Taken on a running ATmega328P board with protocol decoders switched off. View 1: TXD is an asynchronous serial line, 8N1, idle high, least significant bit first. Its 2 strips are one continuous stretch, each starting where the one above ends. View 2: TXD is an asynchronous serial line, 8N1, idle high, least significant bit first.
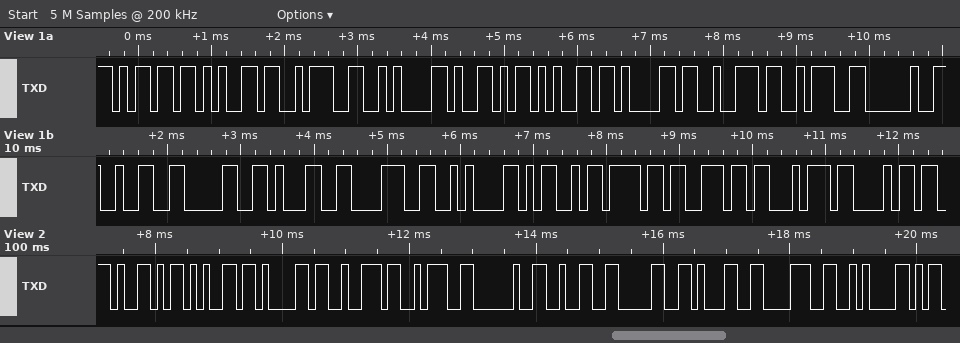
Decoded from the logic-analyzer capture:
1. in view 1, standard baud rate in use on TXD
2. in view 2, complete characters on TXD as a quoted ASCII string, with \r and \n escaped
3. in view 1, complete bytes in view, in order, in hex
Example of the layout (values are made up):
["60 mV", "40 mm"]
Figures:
["9600 baud", "\"Year: 2018\\n\"", "6D 65 3A 0A 59 65 61 72 3A 20 32 30 31 38 0A 4D 6F 6E 74 68"]
